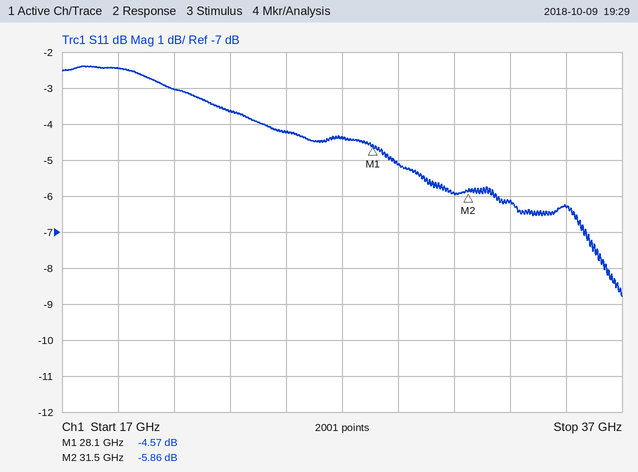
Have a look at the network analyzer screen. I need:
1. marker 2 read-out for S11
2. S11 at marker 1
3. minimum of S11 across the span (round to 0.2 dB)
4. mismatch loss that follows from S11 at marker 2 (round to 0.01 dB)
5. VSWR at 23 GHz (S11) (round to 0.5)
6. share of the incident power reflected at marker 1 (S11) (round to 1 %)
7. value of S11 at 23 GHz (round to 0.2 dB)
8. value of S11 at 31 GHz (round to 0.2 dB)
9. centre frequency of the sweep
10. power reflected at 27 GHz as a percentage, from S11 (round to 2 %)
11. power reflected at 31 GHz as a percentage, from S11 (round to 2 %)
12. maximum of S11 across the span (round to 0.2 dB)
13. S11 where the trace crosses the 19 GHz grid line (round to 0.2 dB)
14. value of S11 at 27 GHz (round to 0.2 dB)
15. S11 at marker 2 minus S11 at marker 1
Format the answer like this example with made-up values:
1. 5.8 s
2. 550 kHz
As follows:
1. -5.86 dB
2. -4.57 dB
3. -8.8 dB
4. 1.30 dB
5. 5.0
6. 35 %
7. -3.6 dB
8. -6.0 dB
9. 27 GHz
10. 36 %
11. 26 %
12. -2.4 dB
13. -2.4 dB
14. -4.4 dB
15. -1.29 dB
